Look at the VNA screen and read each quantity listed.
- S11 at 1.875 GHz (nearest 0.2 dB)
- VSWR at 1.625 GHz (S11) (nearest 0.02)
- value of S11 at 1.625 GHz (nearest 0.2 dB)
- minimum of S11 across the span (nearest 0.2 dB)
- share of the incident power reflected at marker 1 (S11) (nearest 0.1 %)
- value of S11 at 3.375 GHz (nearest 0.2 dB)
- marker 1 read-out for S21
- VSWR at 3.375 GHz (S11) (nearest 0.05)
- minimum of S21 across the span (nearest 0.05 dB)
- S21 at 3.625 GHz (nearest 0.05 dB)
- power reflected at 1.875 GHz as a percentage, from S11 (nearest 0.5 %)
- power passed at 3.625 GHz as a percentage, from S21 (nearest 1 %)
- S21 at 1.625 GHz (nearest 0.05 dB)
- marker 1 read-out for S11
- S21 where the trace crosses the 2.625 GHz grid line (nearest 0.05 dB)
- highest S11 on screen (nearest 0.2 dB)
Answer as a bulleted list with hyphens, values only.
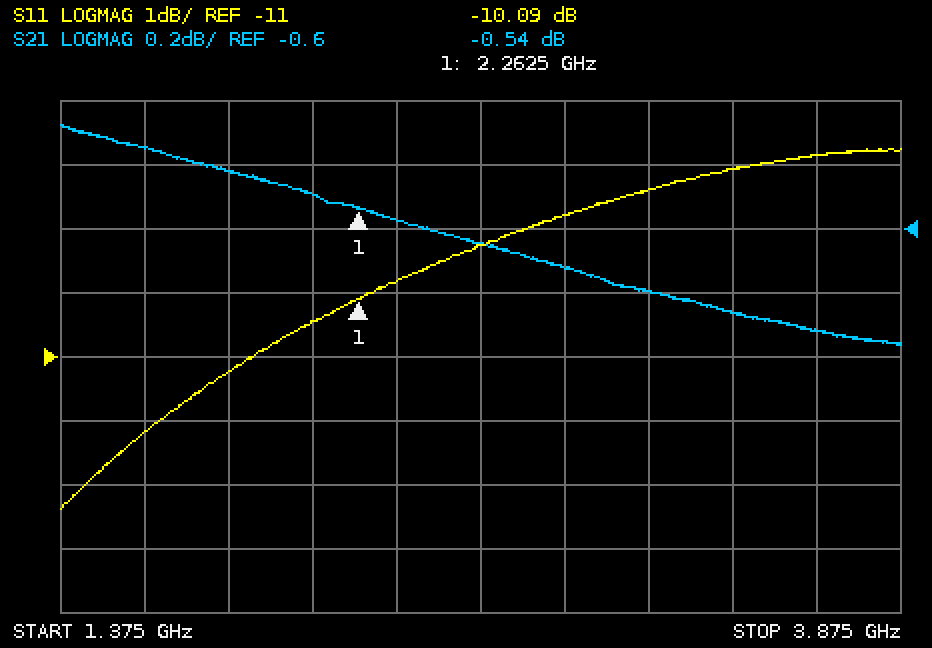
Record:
- -11.2 dB
- 1.66
- -12.2 dB
- -13.4 dB
- 9.8 %
- -8.0 dB
- -0.54 dB
- 2.30
- -0.95 dB
- -0.90 dB
- 7.5 %
- 81 %
- -0.35 dB
- -10.09 dB
- -0.65 dB
- -7.8 dB
